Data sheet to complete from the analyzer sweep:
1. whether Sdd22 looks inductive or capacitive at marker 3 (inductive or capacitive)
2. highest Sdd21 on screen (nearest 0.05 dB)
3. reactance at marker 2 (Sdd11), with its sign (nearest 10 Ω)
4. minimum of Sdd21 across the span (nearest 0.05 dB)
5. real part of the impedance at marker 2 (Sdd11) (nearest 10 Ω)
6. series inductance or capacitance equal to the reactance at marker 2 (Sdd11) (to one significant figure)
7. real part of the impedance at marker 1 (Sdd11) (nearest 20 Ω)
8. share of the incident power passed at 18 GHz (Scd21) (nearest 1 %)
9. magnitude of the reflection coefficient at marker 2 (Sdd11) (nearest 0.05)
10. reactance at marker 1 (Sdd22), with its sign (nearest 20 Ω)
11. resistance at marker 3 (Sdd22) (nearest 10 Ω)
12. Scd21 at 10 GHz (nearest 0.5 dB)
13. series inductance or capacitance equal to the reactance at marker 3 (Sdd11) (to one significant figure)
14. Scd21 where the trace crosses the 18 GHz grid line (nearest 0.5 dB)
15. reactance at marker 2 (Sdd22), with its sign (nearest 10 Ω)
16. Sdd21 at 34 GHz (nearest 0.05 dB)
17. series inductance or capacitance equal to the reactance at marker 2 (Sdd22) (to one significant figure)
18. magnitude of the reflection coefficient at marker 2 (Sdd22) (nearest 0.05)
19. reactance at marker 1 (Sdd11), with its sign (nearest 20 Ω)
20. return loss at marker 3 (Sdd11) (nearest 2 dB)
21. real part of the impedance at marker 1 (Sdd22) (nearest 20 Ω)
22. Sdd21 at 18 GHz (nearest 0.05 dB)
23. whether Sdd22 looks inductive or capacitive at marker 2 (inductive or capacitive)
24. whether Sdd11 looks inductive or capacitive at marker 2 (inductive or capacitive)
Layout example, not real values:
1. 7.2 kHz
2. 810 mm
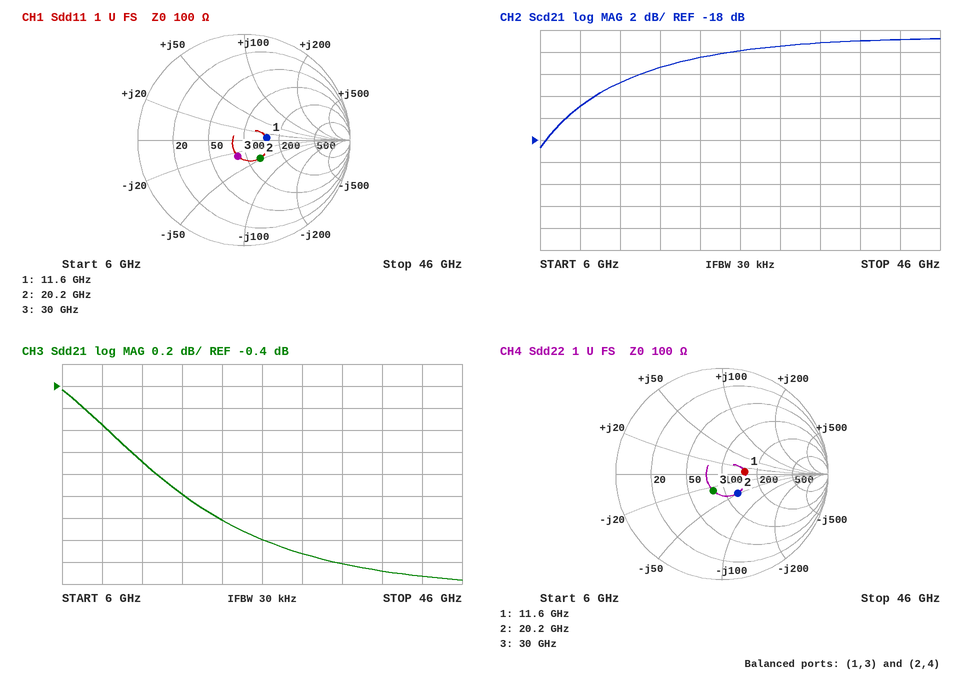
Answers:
1. capacitive
2. -0.45 dB
3. -50 Ω
4. -2.15 dB
5. 130 Ω
6. 200 fF
7. 160 Ω
8. 7 %
9. 0.25
10. 0 Ω
11. 80 Ω
12. -15.0 dB
13. 200 fF
14. -11.5 dB
15. -50 Ω
16. -2.00 dB
17. 200 fF
18. 0.25
19. 0 Ω
20. 16 dB
21. 160 Ω
22. -1.40 dB
23. capacitive
24. capacitive
